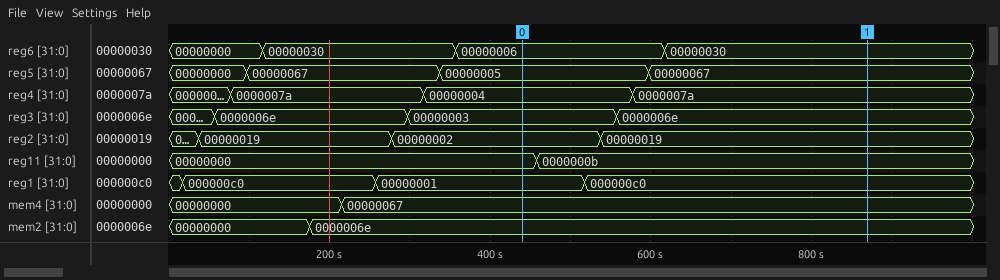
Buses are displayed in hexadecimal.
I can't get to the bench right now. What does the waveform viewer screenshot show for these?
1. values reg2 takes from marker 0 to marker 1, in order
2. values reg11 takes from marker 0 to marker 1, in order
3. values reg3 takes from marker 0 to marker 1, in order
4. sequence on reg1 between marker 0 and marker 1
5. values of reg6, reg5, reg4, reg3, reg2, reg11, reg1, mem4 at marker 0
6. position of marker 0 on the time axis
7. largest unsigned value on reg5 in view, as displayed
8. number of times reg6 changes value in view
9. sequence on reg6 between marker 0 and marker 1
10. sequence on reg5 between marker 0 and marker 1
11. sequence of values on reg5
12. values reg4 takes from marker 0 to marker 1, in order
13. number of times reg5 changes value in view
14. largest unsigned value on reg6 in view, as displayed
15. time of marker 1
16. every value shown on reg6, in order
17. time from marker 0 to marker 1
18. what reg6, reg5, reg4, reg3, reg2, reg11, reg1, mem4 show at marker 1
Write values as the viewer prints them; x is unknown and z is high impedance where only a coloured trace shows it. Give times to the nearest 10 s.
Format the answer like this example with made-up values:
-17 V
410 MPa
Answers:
00000002, 00000019
00000000, 0000000b
00000003, 0000006e
00000001, 000000c0
reg6=00000006, reg5=00000005, reg4=00000004, reg3=00000003, reg2=00000002, reg11=00000000, reg1=00000001, mem4=00000067
440 s
00000067
3
00000006, 00000030
00000005, 00000067
00000000, 00000067, 00000005, 00000067
00000004, 0000007a
3
00000030
870 s
00000000, 00000030, 00000006, 00000030
430 s
reg6=00000030, reg5=00000067, reg4=0000007a, reg3=0000006e, reg2=00000019, reg11=0000000b, reg1=000000c0, mem4=00000067
